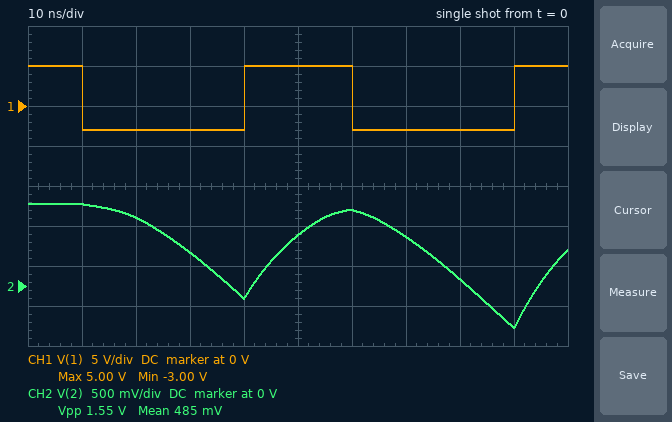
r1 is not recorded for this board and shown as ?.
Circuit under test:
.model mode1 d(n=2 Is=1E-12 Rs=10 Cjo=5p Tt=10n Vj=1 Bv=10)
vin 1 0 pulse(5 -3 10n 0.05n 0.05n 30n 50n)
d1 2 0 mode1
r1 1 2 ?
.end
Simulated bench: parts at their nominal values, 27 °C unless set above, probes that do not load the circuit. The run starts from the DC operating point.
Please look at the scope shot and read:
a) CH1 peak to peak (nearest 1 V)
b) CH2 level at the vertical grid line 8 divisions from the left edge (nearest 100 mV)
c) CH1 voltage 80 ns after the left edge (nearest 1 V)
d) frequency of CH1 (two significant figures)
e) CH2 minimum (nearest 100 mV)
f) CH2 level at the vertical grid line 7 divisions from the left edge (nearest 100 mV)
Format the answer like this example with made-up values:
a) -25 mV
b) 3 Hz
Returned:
a) 8 V
b) 100 mV
c) -3 V
d) 20 MHz
e) -500 mV
f) 600 mV
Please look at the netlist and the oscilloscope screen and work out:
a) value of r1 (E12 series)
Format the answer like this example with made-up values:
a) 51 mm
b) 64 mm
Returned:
a) 10 kΩ
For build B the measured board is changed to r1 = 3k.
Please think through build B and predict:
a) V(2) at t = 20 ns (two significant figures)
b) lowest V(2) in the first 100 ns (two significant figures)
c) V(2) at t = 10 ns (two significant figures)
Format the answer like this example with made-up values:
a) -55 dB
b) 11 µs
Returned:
a) 610 mV
b) -2.6 V
c) 1.1 V
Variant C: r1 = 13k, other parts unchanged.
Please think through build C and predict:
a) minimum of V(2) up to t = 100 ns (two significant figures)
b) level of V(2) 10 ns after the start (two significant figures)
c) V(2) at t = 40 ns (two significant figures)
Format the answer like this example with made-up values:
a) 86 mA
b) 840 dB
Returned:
a) -180 mV
b) 1.0 V
c) 140 mV
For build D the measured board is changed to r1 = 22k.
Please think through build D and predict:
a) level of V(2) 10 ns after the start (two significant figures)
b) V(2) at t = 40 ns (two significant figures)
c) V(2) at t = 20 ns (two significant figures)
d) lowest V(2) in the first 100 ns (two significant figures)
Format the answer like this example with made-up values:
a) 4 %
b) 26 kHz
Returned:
a) 990 mV
b) 500 mV
c) 880 mV
d) 290 mV
